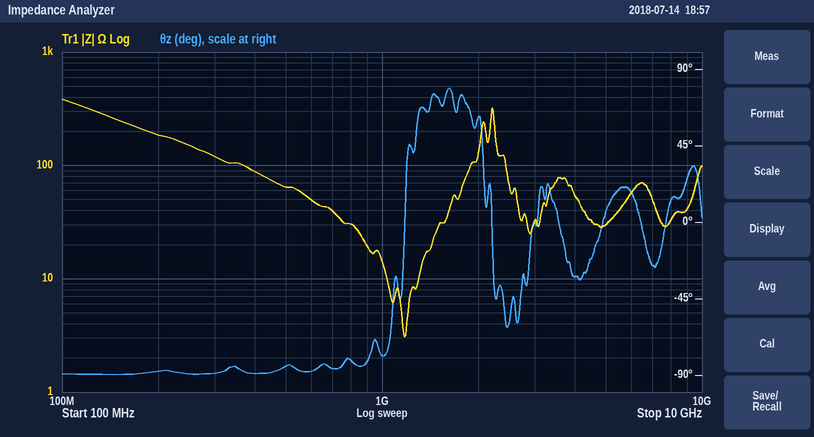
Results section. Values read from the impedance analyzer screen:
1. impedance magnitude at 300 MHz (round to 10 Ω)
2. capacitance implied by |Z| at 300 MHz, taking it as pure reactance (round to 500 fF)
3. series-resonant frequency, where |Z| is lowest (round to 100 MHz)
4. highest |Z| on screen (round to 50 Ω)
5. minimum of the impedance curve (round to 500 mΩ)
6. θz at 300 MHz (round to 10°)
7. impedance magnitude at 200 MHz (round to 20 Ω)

120 Ω
4.5 pF
1.2 GHz
400 Ω
3.0 Ω
-90°
180 Ω
